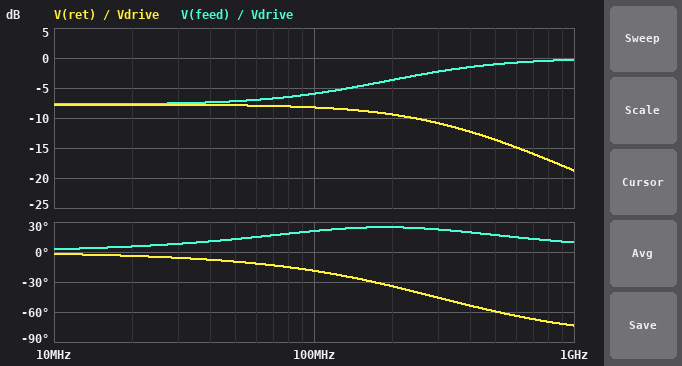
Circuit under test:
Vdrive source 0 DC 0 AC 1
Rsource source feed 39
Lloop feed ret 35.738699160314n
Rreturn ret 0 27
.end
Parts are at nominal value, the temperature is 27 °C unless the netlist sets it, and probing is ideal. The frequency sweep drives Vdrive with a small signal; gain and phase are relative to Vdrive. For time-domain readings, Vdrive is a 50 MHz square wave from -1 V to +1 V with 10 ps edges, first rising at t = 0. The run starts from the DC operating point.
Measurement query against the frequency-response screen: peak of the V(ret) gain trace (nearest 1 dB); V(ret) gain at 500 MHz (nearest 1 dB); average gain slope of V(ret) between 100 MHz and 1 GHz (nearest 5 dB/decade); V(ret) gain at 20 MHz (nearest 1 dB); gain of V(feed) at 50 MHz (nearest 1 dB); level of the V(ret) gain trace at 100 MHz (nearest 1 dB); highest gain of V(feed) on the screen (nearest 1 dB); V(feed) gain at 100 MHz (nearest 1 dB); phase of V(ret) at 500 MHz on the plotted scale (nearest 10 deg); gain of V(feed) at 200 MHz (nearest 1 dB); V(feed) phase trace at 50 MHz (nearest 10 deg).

-8 dB
-14 dB
-10 dB/decade
-8 dB
-7 dB
-8 dB
0 dB
-6 dB
-60 deg
-4 dB
10 deg
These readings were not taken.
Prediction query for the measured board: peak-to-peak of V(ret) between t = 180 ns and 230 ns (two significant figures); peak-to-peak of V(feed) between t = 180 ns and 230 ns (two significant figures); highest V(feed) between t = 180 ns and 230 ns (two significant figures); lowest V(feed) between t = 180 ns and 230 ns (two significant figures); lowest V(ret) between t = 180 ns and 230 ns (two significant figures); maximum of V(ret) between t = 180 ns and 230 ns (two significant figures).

820 mV
3.2 V
1.6 V
-1.6 V
-410 mV
410 mV
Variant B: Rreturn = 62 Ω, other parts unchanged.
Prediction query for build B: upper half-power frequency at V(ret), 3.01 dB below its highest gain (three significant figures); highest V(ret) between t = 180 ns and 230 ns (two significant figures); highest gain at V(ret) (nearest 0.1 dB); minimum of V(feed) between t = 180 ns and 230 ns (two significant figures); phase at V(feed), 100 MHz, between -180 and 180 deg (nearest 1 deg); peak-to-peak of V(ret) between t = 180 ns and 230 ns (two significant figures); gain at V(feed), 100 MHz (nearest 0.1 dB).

450 MHz
610 mV
-4.2 dB
-1.4 V
7 deg
1.2 V
-3.9 dB
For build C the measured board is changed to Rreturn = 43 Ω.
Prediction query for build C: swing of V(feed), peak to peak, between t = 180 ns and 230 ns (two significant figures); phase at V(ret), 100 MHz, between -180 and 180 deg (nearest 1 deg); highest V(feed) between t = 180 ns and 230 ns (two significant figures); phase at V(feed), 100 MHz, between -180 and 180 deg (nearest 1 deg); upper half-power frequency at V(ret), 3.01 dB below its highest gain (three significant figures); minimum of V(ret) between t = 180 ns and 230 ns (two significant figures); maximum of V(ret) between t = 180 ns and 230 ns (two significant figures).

2.9 V
-15 deg
1.5 V
12 deg
365 MHz
-520 mV
520 mV
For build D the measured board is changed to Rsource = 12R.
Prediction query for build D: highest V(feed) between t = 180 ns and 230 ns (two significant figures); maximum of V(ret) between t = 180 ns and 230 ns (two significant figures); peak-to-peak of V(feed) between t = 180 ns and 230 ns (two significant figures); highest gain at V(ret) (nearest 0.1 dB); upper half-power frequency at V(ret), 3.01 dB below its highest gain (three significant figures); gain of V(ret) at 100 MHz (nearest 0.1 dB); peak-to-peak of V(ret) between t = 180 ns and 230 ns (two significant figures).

1.3 V
690 mV
2.6 V
-3.2 dB
174 MHz
-4.4 dB
1.4 V
